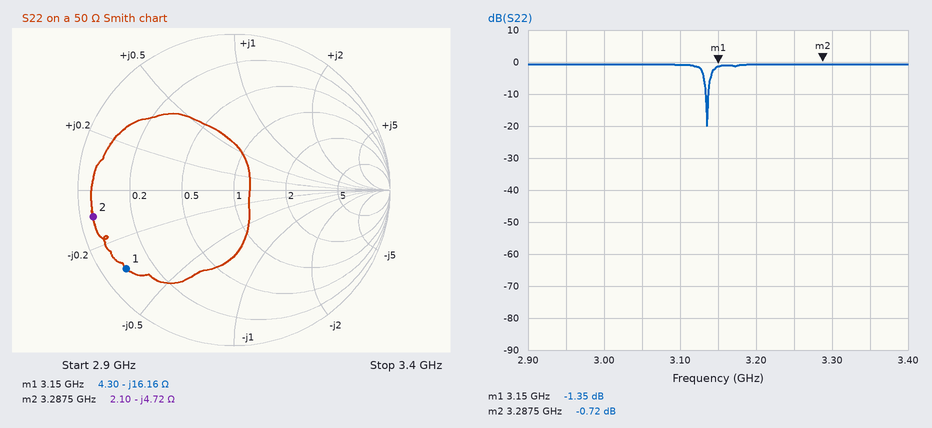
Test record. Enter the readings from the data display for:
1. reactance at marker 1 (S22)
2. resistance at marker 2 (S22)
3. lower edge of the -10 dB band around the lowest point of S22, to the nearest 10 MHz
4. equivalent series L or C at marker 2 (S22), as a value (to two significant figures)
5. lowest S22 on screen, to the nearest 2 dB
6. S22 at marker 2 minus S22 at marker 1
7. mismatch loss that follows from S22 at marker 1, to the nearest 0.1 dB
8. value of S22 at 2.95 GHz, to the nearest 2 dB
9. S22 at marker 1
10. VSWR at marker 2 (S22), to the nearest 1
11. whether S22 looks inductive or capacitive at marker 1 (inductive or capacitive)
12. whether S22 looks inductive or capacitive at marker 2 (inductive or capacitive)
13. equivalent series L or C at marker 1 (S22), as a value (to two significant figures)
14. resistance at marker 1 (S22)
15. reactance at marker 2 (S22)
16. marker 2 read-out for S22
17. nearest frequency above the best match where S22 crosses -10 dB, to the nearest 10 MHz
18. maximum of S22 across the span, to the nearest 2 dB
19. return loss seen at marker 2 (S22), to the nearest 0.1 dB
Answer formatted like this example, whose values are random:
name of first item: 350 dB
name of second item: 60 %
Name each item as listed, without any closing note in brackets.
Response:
reactance at marker 1: -16.16 Ω
resistance at marker 2: 2.10 Ω
lower edge of the -10 dB band around the lowest point of S22, to the nearest 10 MHz: 3.13 GHz
equivalent series L or C at marker 2 (S22), as a value: 10 pF
lowest S22 on screen, to the nearest 2 dB: -20 dB
S22 at marker 2 minus S22 at marker 1: 0.63 dB
mismatch loss that follows from S22 at marker 1, to the nearest 0.1 dB: 5.7 dB
value of S22 at 2.95 GHz, to the nearest 2 dB: 0 dB
S22 at marker 1: -1.35 dB
VSWR at marker 2 (S22), to the nearest 1: 24
whether S22 looks inductive or capacitive at marker 1: capacitive
whether S22 looks inductive or capacitive at marker 2: capacitive
equivalent series L or C at marker 1 (S22), as a value: 3.1 pF
resistance at marker 1: 4.30 Ω
reactance at marker 2: -4.72 Ω
marker 2 read-out for S22: -0.72 dB
nearest frequency above the best match where S22 crosses -10 dB, to the nearest 10 MHz: 3.14 GHz
maximum of S22 across the span, to the nearest 2 dB: 0 dB
return loss seen at marker 2 (S22), to the nearest 0.1 dB: 0.7 dB
